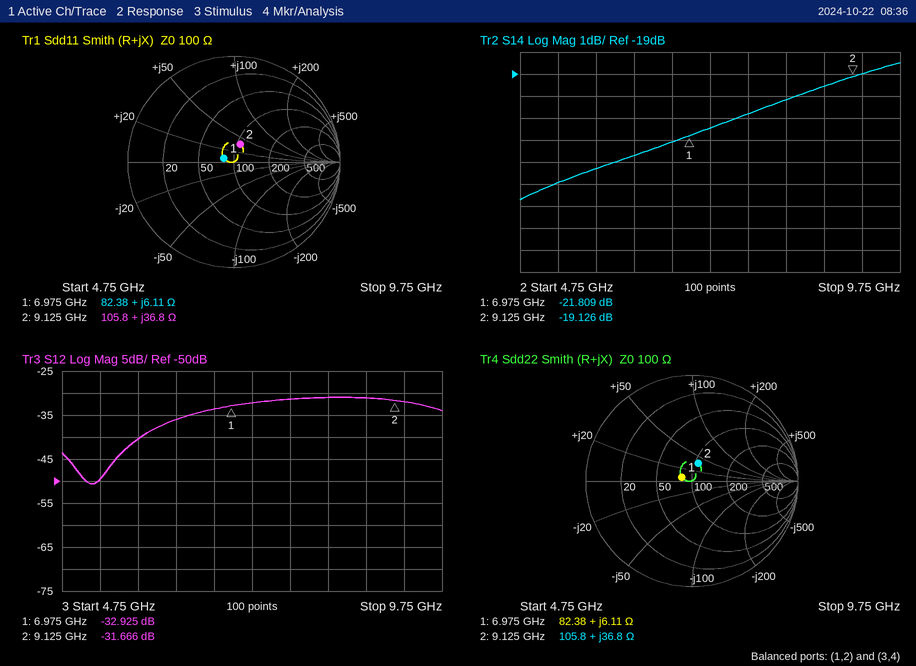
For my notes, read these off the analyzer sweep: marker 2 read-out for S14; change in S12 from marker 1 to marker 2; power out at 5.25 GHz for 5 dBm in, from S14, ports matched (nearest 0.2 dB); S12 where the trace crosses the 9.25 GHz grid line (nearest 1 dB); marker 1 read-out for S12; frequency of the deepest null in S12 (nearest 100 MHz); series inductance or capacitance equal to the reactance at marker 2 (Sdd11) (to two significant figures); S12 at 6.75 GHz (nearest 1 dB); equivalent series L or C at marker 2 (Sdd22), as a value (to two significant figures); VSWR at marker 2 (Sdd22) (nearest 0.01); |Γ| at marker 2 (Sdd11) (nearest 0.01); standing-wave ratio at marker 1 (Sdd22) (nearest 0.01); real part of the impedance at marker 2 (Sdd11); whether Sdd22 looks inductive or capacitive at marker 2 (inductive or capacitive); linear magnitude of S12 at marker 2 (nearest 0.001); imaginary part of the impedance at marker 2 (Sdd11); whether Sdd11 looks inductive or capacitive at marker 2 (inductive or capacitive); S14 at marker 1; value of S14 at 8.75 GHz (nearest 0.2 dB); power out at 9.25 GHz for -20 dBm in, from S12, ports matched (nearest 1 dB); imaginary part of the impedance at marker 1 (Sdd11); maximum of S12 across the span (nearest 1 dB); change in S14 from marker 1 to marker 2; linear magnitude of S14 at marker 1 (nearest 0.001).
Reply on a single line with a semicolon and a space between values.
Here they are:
-19.126 dB; 1.259 dB; -19.0 dBm; -32 dB; -32.925 dB; 5.1 GHz; 640 pH; -34 dB; 640 pH; 1.43; 0.18; 1.23; 105.8 Ω; inductive; 0.026; +36.8 Ω; inductive; -21.809 dB; -19.6 dB; -52 dBm; +6.11 Ω; -31 dB; 2.683 dB; 0.081
